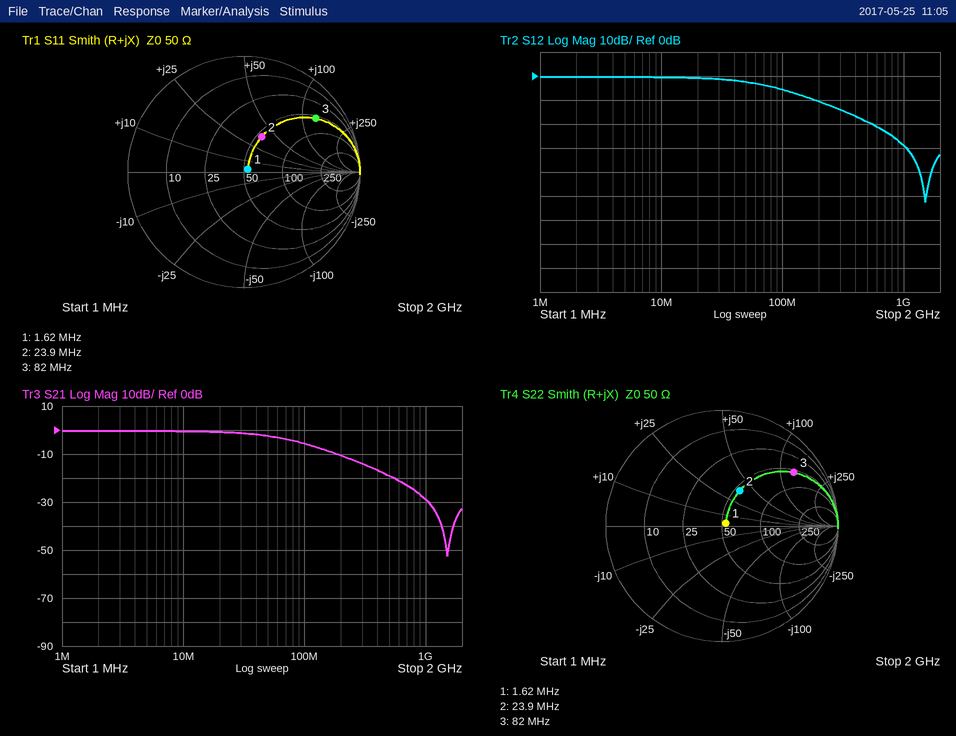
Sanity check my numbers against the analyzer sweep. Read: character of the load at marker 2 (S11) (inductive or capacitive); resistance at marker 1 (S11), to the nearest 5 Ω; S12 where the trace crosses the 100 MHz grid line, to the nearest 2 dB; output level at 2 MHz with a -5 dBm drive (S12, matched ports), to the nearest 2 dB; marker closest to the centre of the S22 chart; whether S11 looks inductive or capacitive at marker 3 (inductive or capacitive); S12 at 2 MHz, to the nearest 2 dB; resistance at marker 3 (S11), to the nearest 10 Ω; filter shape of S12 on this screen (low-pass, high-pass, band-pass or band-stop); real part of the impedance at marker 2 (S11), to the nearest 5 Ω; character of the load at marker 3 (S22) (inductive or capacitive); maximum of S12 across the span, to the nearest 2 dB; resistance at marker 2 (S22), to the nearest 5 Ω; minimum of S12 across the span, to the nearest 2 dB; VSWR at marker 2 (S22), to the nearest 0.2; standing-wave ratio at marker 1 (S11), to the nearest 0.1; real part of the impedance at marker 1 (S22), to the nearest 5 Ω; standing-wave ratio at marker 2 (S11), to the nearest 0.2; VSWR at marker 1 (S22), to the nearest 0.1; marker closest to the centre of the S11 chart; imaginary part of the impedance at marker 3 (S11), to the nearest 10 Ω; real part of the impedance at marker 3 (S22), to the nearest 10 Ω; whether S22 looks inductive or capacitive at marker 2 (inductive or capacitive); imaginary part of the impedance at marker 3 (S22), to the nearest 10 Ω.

inductive
55 Ω
-6 dB
-6 dBm
marker 1
inductive
0 dB
60 Ω
low-pass
55 Ω
inductive
0 dB
55 Ω
-52 dB
2.0
1.1
55 Ω
2.0
1.1
marker 1
+130 Ω
60 Ω
inductive
+130 Ω
